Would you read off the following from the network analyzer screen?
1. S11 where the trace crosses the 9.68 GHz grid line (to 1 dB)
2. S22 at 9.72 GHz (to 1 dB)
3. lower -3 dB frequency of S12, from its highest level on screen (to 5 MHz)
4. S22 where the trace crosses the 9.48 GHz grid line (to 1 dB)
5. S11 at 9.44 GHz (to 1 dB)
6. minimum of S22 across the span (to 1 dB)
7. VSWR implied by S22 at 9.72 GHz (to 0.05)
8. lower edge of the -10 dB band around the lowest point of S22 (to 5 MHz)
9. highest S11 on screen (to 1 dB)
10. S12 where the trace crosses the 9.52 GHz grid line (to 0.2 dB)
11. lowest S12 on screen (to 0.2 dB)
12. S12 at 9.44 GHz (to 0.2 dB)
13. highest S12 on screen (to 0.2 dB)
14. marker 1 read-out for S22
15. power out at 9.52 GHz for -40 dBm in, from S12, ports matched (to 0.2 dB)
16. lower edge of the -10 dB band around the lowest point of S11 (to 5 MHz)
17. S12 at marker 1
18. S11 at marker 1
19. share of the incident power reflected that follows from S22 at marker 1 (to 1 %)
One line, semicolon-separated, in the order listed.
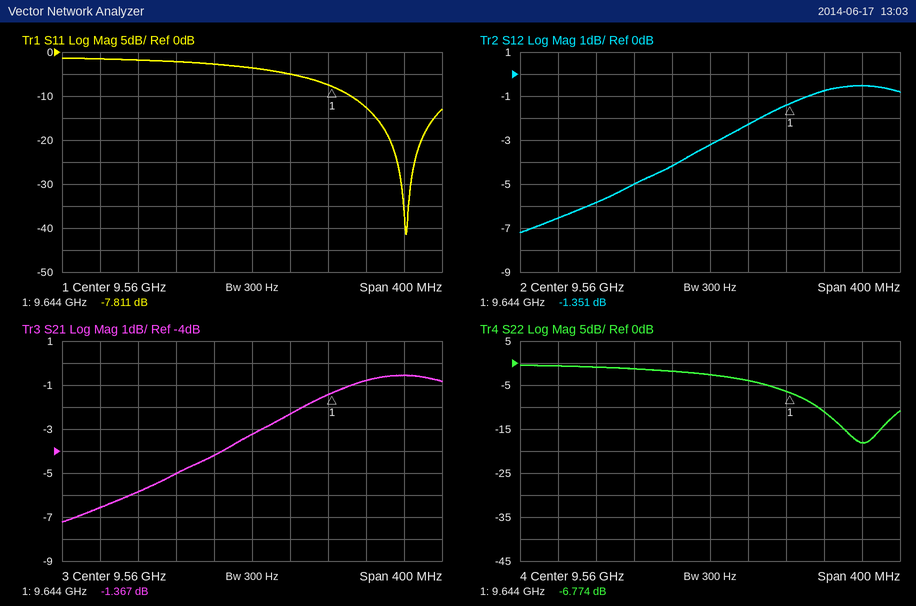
-13 dB; -18 dB; 9.545 GHz; -1 dB; -2 dB; -18 dB; 1.30; 9.675 GHz; -1 dB; -4.2 dB; -7.2 dB; -5.8 dB; -0.6 dB; -6.774 dB; -44.2 dBm; 9.665 GHz; -1.351 dB; -7.811 dB; 21 %
